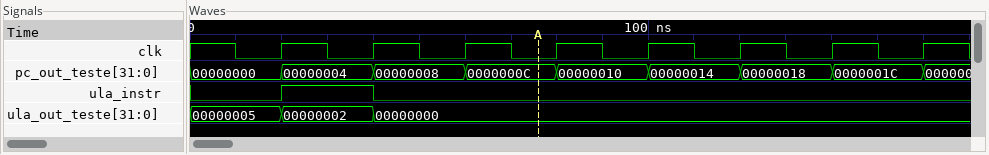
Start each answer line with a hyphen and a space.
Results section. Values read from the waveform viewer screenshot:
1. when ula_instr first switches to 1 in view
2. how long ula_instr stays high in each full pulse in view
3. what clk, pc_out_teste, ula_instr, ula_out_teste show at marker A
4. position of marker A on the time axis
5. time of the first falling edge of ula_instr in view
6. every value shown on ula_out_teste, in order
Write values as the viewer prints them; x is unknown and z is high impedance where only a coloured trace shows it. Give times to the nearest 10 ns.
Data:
- 20 ns
- 20 ns
- clk=0, pc_out_teste=0000000C, ula_instr=0, ula_out_teste=00000000
- 80 ns
- 40 ns
- 00000005, 00000002, 00000000
